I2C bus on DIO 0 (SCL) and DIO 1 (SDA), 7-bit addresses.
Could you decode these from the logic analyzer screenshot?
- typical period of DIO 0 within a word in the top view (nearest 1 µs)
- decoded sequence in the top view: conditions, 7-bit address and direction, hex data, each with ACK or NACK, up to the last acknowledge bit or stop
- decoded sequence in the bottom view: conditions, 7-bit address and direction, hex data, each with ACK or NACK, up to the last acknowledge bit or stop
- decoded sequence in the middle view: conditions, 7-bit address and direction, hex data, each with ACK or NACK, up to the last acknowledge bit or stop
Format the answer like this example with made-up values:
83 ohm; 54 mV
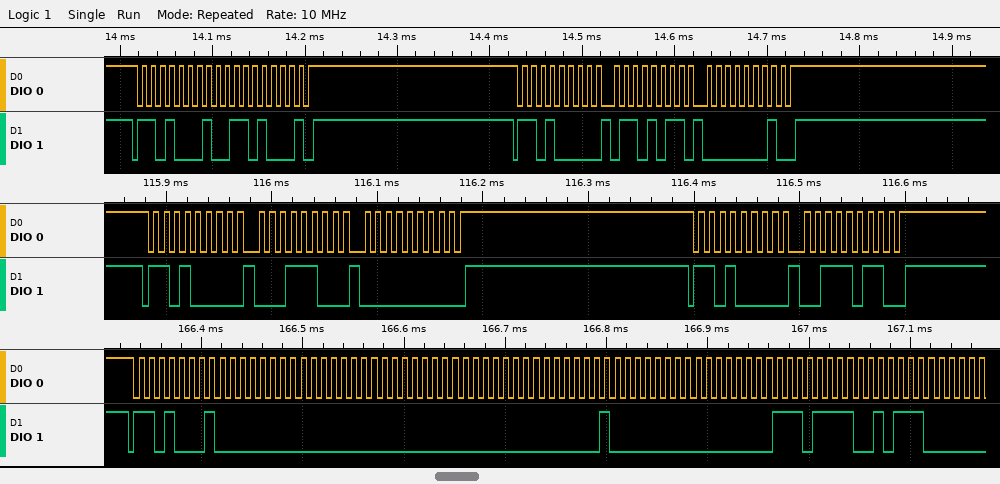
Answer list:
10 µs; start, address 68 read ACK, 68 NACK, stop, start, address 68 write ACK, 6B ACK, 01 ACK, stop; start, address 68 read ACK, 00 ACK, 00 ACK, 00 ACK, 00 ACK, 40 ACK, 00 ACK, EF ACK, 5C ACK; start, address 68 write ACK, 1C ACK, 00 ACK, stop, start, address 68 write ACK, 3B ACK, stop
